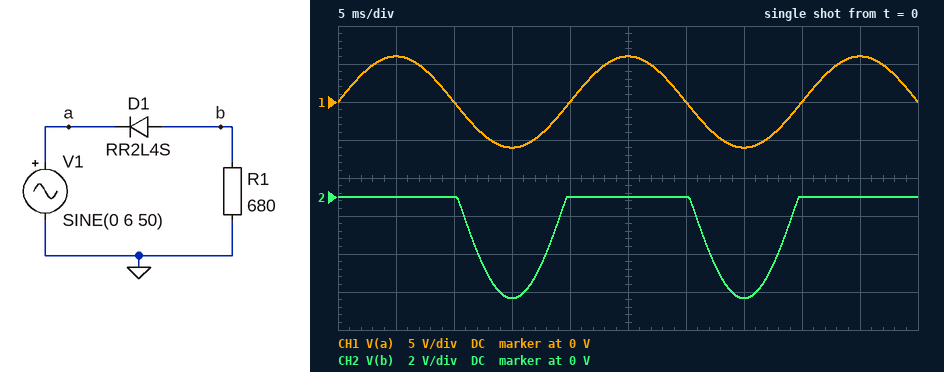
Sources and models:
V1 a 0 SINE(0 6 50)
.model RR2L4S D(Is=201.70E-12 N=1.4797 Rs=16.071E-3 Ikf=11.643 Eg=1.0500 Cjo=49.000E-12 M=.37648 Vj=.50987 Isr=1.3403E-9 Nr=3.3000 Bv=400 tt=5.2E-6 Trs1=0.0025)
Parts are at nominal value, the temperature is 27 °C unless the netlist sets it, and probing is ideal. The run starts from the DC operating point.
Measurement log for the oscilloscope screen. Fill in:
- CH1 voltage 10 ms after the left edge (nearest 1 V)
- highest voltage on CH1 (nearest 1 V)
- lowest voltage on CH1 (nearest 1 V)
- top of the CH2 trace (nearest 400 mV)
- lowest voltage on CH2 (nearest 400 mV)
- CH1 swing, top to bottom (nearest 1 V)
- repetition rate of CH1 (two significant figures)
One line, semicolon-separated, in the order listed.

0 V; 6 V; -6 V; 0 V; -5.2 V; 12 V; 50 Hz
